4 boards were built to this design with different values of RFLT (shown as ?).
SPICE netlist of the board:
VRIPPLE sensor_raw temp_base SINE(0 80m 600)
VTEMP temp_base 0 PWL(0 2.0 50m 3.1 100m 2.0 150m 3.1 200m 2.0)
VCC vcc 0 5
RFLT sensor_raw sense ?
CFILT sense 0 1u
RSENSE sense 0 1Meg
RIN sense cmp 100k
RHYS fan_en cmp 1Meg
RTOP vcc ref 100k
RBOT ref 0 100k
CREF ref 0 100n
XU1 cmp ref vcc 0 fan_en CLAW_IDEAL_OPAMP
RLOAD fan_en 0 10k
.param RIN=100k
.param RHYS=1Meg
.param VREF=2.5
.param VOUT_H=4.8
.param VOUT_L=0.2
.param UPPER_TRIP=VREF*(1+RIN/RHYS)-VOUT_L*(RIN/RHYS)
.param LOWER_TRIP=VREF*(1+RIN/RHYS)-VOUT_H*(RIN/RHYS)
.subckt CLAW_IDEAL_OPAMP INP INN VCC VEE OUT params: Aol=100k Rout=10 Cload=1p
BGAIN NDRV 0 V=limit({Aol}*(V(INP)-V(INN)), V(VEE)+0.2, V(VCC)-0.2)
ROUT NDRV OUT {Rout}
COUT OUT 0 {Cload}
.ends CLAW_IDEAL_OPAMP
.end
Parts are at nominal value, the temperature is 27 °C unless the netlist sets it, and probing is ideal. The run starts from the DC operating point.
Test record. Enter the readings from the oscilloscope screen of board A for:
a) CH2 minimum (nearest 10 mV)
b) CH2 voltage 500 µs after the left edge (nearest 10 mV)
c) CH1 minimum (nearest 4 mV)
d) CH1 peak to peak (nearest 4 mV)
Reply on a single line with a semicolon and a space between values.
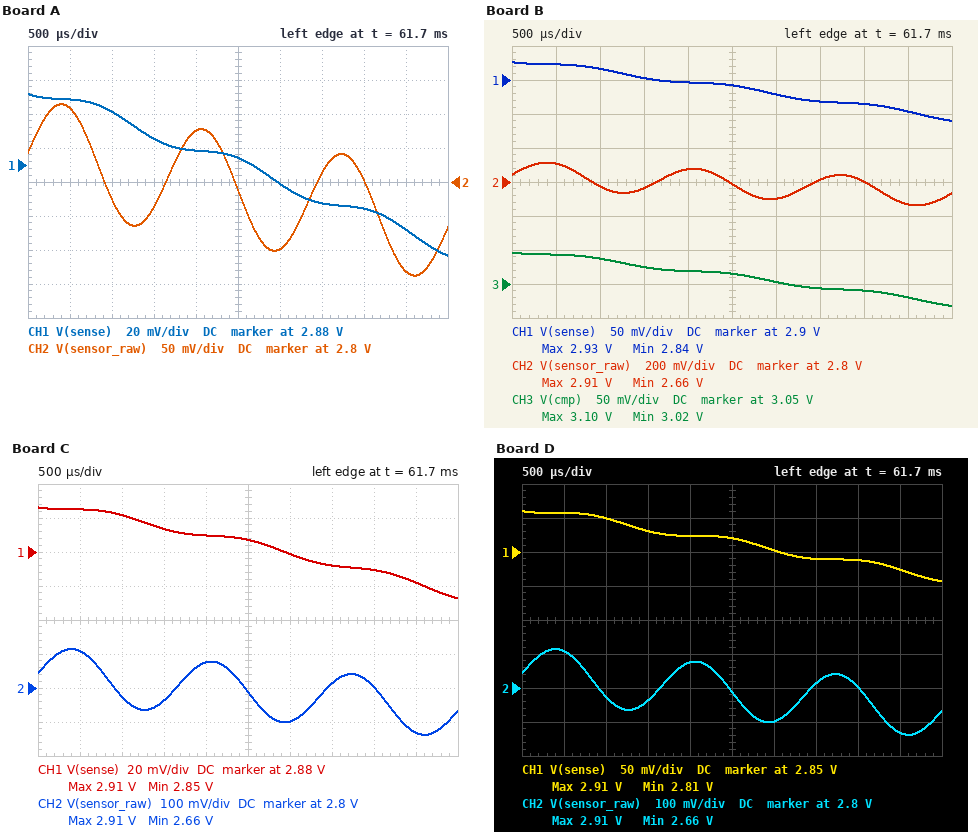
2.66 V; 2.91 V; 2.828 V; 96 mV
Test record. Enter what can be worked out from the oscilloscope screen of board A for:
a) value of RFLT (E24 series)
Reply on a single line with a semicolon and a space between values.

5.1 kΩ
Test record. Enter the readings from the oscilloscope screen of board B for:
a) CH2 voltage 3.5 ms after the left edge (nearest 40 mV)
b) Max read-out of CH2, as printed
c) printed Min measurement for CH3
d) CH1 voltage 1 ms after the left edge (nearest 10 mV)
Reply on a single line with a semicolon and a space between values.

2.80 V; 2.91 V; 3.02 V; 2.92 V
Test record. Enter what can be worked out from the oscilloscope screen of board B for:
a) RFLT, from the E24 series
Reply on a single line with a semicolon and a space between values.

6.2 kΩ
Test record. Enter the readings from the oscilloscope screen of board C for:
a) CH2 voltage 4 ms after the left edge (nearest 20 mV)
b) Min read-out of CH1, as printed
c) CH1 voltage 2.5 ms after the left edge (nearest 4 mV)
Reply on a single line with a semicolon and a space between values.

2.80 V; 2.85 V; 2.888 V
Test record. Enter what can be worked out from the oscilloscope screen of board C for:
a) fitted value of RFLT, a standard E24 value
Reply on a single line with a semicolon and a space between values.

10 kΩ
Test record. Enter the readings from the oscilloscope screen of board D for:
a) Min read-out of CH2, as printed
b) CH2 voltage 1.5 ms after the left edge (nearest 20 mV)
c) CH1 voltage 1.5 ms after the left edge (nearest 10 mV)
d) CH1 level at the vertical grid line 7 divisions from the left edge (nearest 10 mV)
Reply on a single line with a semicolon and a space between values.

2.66 V; 2.76 V; 2.88 V; 2.84 V
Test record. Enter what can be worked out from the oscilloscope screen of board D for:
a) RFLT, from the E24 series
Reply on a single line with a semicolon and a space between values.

3.9 kΩ
